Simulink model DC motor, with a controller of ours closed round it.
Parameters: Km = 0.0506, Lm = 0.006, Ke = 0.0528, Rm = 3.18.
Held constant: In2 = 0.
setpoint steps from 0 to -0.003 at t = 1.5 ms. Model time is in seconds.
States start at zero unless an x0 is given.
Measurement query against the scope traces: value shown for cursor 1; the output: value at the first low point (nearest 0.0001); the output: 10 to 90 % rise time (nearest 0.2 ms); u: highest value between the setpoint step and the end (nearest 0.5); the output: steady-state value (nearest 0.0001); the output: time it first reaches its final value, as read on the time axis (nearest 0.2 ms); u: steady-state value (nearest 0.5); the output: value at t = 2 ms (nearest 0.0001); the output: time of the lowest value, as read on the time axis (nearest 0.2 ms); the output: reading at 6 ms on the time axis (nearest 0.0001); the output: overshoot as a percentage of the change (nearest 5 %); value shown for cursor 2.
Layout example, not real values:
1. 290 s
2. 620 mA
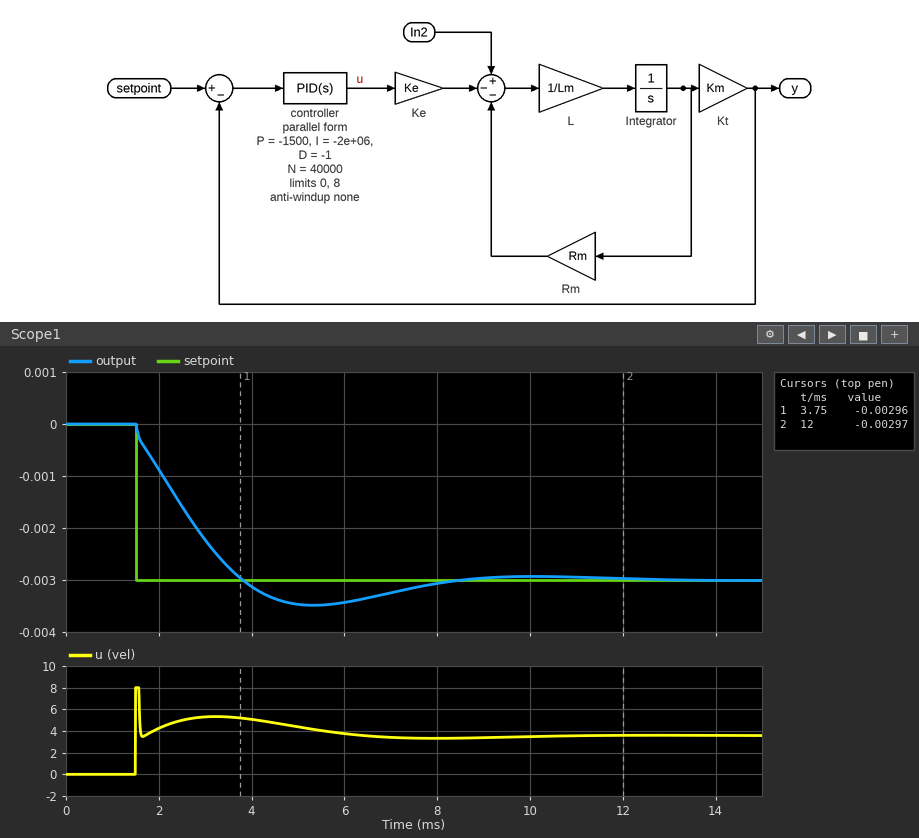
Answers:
1. -0.00296
2. -0.0035
3. 1.8 ms
4. 8.0
5. -0.0030
6. 3.8 ms
7. 3.5
8. -0.0009
9. 5.4 ms
10. -0.0034
11. 15 %
12. -0.00297
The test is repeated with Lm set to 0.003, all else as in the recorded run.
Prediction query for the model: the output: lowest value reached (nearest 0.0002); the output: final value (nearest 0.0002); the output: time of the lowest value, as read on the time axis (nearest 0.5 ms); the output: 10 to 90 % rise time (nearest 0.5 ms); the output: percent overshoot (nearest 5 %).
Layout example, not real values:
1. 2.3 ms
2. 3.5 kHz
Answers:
1. -0.0032
2. -0.0030
3. 5.0 ms
4. 1.5 ms
5. 10 %
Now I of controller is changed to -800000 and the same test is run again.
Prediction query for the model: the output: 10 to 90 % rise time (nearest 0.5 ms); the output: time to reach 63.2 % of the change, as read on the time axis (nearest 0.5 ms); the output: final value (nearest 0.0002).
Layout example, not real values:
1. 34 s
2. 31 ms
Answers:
1. 3.5 ms
2. 3.5 ms
3. -0.0030
